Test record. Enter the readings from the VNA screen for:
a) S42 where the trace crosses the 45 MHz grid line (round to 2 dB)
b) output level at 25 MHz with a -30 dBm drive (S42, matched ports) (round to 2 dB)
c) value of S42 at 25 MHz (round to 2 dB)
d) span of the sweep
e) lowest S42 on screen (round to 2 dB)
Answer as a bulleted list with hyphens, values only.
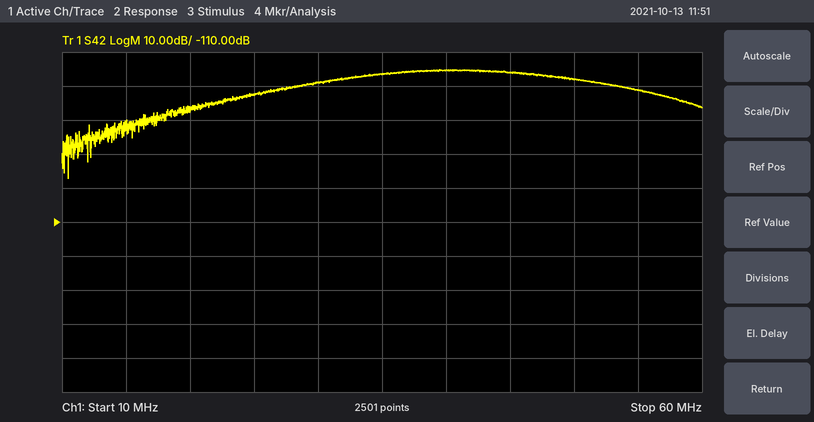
- -66 dB
- -102 dBm
- -72 dB
- 50 MHz
- -98 dB
